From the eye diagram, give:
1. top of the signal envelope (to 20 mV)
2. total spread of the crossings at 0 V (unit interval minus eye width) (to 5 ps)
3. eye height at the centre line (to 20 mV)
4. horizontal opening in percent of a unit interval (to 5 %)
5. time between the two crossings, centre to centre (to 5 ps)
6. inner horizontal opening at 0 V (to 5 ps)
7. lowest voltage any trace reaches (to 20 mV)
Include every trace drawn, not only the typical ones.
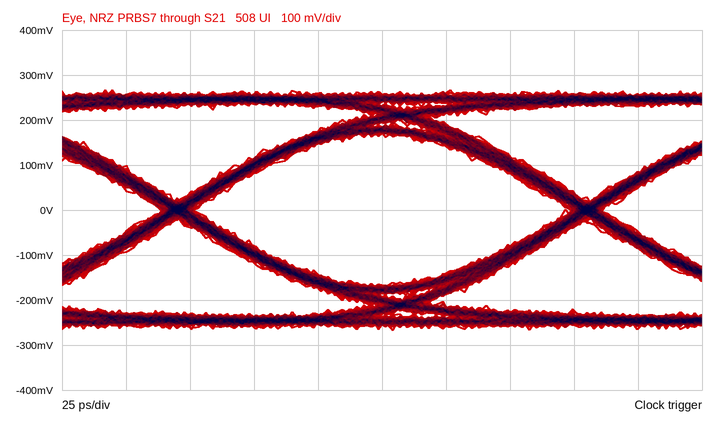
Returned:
260 mV
15 ps
340 mV
90 %
160 ps
145 ps
-260 mV
